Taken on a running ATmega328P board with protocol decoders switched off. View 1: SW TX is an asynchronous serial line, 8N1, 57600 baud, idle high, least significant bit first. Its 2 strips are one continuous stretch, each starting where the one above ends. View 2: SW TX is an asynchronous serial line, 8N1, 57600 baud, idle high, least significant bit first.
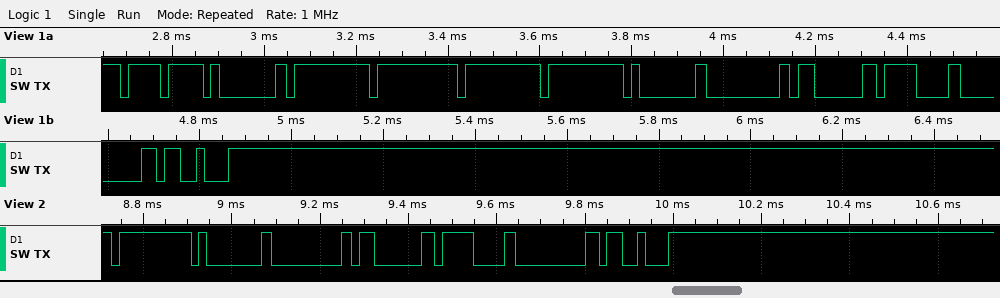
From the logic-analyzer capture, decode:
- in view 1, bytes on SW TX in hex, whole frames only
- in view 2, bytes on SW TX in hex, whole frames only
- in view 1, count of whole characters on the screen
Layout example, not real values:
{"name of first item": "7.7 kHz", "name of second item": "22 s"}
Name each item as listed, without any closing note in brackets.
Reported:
{"in view 1, bytes on SW TX in hex, whole frames only": "0xEF 0x01 0xFF 0xFF 0xFF 0xFF 0x01 0x00 0x03 0x0F 0x00 0x13", "in view 2, bytes on SW TX in hex, whole frames only": "FF 01 00 03 0F 00 13", "in view 1, count of whole characters on the screen": "12"}
